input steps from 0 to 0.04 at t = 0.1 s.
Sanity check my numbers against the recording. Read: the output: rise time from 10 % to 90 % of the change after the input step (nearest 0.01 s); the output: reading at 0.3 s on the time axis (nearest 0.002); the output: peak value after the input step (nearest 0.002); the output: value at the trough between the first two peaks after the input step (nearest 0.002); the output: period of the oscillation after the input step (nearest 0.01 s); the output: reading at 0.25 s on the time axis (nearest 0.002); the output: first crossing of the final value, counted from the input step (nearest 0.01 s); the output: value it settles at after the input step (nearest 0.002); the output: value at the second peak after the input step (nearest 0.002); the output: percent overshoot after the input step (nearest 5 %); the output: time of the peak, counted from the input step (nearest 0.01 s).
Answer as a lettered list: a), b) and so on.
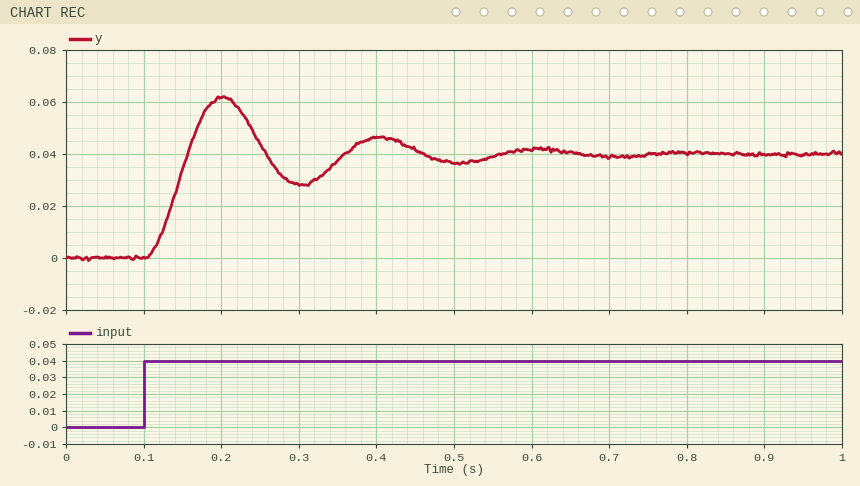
a) 0.04 s
b) 0.028
c) 0.062
d) 0.028
e) 0.20 s
f) 0.044
g) 0.06 s
h) 0.040
i) 0.046
j) 55 %
k) 0.10 s
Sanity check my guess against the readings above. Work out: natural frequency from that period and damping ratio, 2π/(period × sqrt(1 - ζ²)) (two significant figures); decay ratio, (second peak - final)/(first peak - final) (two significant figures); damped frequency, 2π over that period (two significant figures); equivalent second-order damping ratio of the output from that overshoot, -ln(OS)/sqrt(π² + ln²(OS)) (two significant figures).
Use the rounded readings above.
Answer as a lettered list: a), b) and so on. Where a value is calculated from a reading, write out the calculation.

a) 2π / (0.2 × sqrt(1 - 0.19²)) = 32 rad/s
b) (0.046 - 0.04) / (0.062 - 0.04) = 0.27
c) 2π / 0.2 = 31 rad/s
d) ln(0.55) = -0.598; 0.598 / sqrt(9.870 + 0.357) = 0.19
